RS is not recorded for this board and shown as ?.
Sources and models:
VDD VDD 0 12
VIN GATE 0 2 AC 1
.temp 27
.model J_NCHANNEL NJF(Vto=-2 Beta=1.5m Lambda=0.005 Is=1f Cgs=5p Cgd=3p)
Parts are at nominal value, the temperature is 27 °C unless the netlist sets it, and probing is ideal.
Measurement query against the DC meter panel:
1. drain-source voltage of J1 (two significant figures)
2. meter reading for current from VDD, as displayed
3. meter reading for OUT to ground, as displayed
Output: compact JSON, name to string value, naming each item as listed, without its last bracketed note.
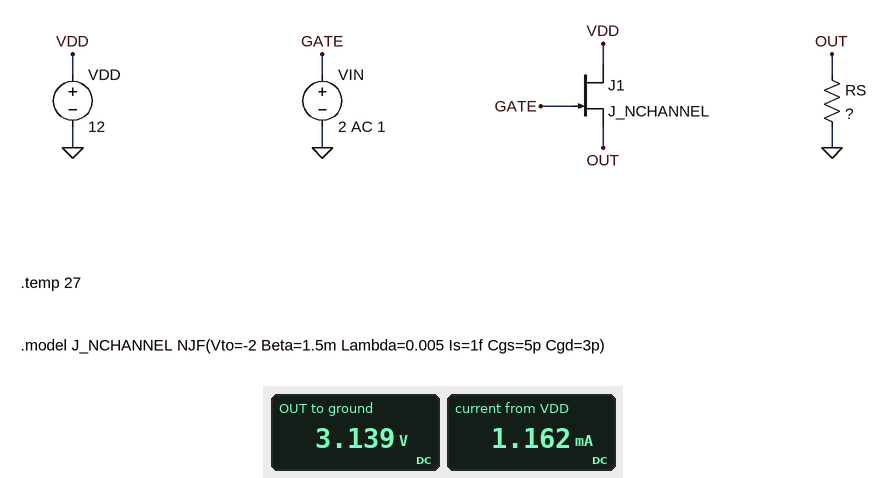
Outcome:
{"drain-source voltage of J1": "8.9 V", "meter reading for current from VDD, as displayed": "1.162 mA", "meter reading for OUT to ground, as displayed": "3.139 V"}
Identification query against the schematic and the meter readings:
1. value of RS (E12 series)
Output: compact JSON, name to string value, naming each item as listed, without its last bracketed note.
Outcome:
{"value of RS": "2.7 kΩ"}
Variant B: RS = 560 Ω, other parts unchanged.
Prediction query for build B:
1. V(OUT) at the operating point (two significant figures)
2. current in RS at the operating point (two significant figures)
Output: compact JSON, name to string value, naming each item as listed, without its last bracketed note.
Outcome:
{"V(OUT) at the operating point": "2.4 V", "current in RS at the operating point": "4.2 mA"}
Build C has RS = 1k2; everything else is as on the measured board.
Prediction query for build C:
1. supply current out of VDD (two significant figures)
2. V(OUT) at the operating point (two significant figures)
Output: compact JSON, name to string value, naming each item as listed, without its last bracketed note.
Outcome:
{"supply current out of VDD": "2.3 mA", "V(OUT) at the operating point": "2.8 V"}
